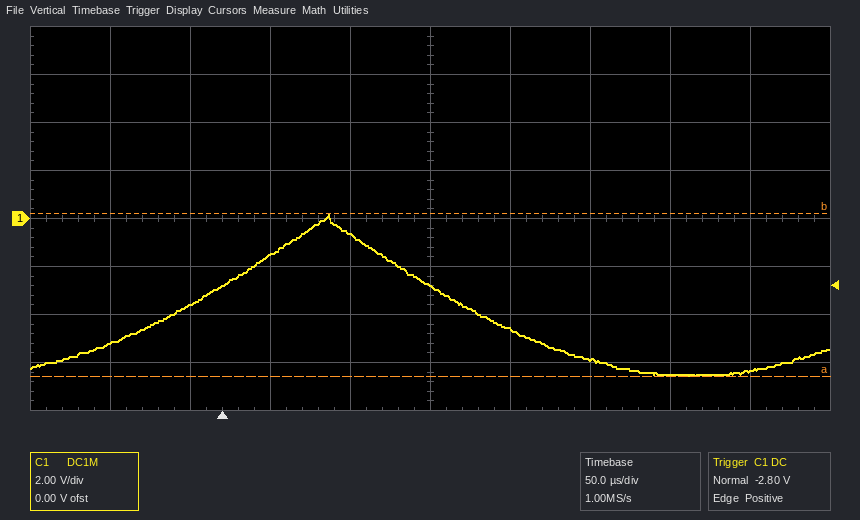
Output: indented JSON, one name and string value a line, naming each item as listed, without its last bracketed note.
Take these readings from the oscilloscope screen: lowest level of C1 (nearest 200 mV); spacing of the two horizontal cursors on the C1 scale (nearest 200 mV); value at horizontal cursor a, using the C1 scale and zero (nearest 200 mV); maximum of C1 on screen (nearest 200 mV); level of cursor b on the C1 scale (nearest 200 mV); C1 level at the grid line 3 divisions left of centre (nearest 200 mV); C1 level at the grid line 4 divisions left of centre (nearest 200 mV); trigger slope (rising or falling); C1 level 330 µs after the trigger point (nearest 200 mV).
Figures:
{
  "lowest level of C1": "-6.6 V",
  "spacing of the two horizontal cursors on the C1 scale": "6.8 V",
  "value at horizontal cursor a, using the C1 scale and zero": "-6.6 V",
  "maximum of C1 on screen": "200 mV",
  "level of cursor b on the C1 scale": "200 mV",
  "C1 level at the grid line 3 divisions left of centre": "-3.6 V",
  "C1 level at the grid line 4 divisions left of centre": "-5.2 V",
  "trigger slope": "rising",
  "C1 level 330 µs after the trigger point": "-6.4 V"
}
